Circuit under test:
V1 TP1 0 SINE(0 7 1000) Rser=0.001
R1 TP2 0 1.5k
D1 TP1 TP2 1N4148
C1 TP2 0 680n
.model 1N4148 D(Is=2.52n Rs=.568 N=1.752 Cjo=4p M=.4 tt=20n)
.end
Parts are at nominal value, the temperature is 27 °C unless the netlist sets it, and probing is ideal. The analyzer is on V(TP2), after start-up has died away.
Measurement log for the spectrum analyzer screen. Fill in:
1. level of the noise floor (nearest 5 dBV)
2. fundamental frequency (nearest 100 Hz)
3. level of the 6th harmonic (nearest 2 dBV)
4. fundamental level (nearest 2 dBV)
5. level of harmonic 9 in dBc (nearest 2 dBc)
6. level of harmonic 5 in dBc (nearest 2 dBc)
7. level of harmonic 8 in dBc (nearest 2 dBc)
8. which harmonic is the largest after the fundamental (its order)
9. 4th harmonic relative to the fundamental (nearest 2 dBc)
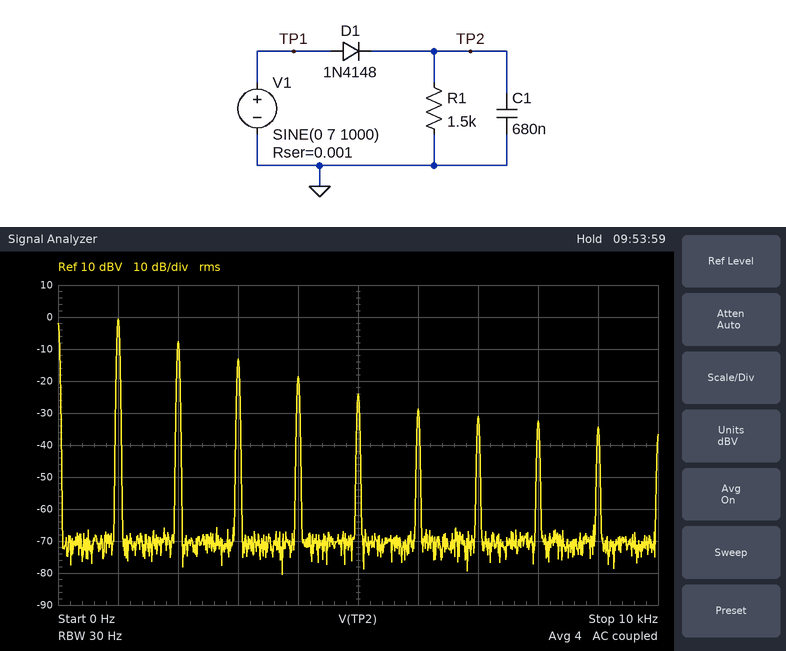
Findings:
-70 dBV
1.0 kHz
-28 dBV
0 dBV
-34 dBc
-24 dBc
-32 dBc
2
-18 dBc
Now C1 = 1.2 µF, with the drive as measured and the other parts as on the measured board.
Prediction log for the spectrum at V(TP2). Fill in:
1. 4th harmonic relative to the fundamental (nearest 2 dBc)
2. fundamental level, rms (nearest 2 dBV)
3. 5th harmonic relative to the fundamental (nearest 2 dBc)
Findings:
-16 dBc
-4 dBV
-20 dBc
